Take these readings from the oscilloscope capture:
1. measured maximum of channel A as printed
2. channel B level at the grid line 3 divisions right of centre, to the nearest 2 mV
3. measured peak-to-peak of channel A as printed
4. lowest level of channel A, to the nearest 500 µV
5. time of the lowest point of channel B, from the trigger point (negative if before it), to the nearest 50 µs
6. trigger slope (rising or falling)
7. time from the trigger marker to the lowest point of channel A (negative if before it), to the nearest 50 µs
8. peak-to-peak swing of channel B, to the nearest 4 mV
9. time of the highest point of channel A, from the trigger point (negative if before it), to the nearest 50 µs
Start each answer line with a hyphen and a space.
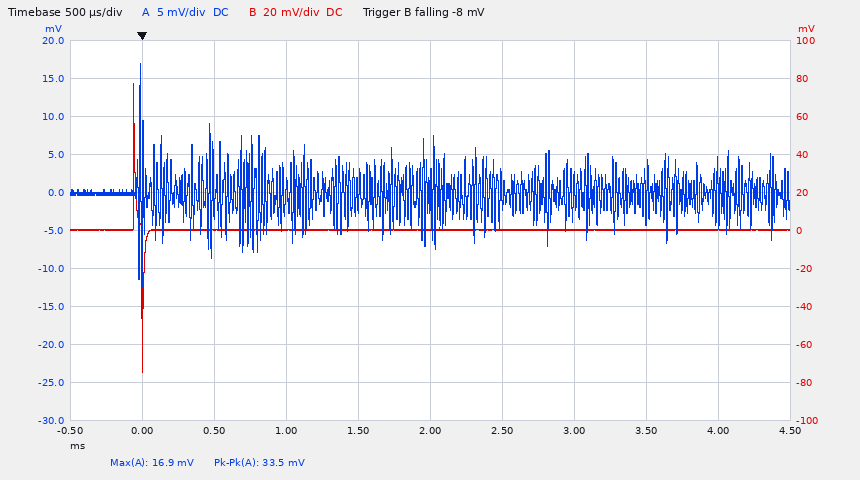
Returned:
- 16.9 mV
- 0 mV
- 33.5 mV
- -16.5 mV
- 0 µs
- falling
- 0 µs
- 152 mV
- 0 µs
